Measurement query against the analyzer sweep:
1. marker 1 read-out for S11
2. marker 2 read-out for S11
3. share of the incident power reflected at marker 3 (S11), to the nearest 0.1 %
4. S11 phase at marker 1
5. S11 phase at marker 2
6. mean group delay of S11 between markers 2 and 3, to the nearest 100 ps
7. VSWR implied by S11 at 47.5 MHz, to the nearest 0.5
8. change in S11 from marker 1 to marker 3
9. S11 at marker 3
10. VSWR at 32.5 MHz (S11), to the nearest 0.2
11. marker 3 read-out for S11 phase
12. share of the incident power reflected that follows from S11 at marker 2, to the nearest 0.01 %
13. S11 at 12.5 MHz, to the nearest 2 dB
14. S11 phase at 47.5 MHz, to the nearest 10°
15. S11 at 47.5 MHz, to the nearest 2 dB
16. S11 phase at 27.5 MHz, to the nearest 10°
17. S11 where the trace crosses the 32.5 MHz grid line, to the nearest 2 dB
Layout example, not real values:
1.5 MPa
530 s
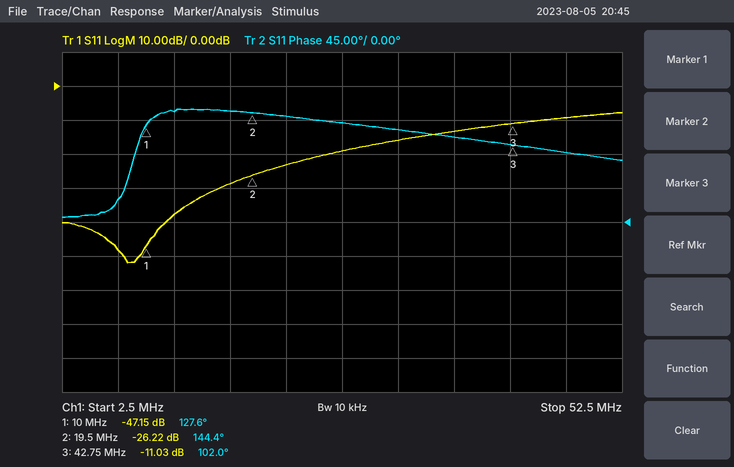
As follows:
-47.15 dB
-26.22 dB
7.9 %
127.6°
144.4°
5.1 ns
2.0
36.12 dB
-11.03 dB
1.4
102.0°
0.24 %
-38 dB
90°
-10 dB
130°
-16 dB
